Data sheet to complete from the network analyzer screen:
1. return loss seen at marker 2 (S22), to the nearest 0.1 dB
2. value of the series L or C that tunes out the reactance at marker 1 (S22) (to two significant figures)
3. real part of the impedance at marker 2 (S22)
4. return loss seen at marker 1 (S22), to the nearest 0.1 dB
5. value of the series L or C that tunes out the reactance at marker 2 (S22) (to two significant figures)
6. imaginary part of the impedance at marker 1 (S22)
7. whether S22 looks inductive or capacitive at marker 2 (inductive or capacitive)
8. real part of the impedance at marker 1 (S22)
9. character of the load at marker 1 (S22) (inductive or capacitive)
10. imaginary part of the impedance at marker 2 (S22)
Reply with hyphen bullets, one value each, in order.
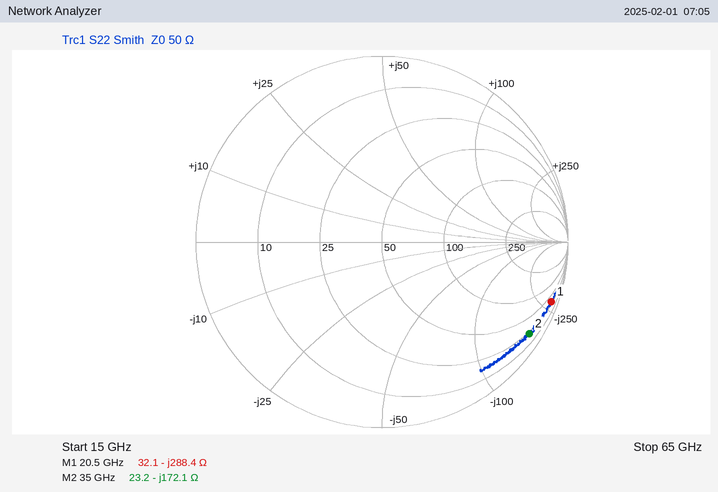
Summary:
- 0.6 dB
- 2.2 nH
- 23.2 Ω
- 0.3 dB
- 780 pH
- -288.4 Ω
- capacitive
- 32.1 Ω
- capacitive
- -172.1 Ω
